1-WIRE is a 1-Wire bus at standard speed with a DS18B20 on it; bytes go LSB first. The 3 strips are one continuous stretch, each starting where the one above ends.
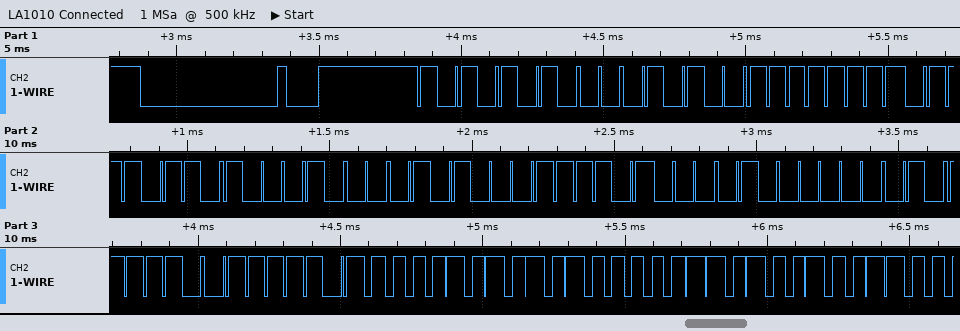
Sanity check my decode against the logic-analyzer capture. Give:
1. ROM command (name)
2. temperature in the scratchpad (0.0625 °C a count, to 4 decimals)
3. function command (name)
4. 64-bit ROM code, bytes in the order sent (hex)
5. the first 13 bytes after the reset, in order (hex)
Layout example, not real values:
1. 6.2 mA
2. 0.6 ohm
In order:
1. Match ROM
2. 85.0000 °C
3. Read Scratchpad
4. 28 FF 6E 11 8A 17 02 7A
5. 55 28 FF 6E 11 8A 17 02 7A BE 50 05 4B
